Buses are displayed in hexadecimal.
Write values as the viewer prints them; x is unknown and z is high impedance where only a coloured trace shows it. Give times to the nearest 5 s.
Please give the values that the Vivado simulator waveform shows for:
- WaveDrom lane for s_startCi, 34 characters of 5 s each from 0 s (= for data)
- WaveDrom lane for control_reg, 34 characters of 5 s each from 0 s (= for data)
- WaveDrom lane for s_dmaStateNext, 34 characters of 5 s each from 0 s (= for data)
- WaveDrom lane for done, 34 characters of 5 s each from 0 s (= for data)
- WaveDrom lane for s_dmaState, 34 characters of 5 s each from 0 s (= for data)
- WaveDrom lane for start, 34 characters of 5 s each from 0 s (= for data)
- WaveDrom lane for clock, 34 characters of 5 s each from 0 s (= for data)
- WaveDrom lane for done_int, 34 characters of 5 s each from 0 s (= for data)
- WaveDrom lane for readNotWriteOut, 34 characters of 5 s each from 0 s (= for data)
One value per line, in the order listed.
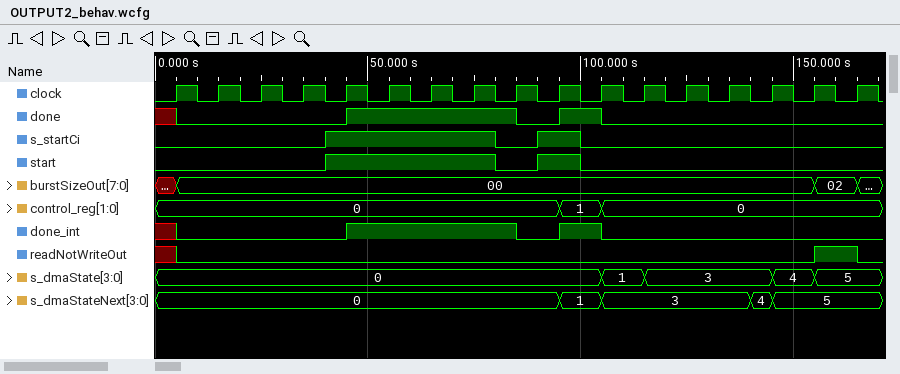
{name: 's_startCi', wave: '0.......1.......0.1.0.............'}
{name: 'control_reg', wave: '=..................=.=............', data: '0 1 0'}
{name: 's_dmaStateNext', wave: '=..................=.=......==....', data: '0 1 3 4 5'}
{name: 'done', wave: 'x0.......1.......0.1.0............'}
{name: 's_dmaState', wave: '=....................=.=.....=.=..', data: '0 1 3 4 5'}
{name: 'start', wave: '0.......1.......0.1.0.............'}
{name: 'clock', wave: '0101010101010101010101010101010101'}
{name: 'done_int', wave: 'x0.......1.......0.1.0............'}
{name: 'readNotWriteOut', wave: 'x0.............................1.0'}
